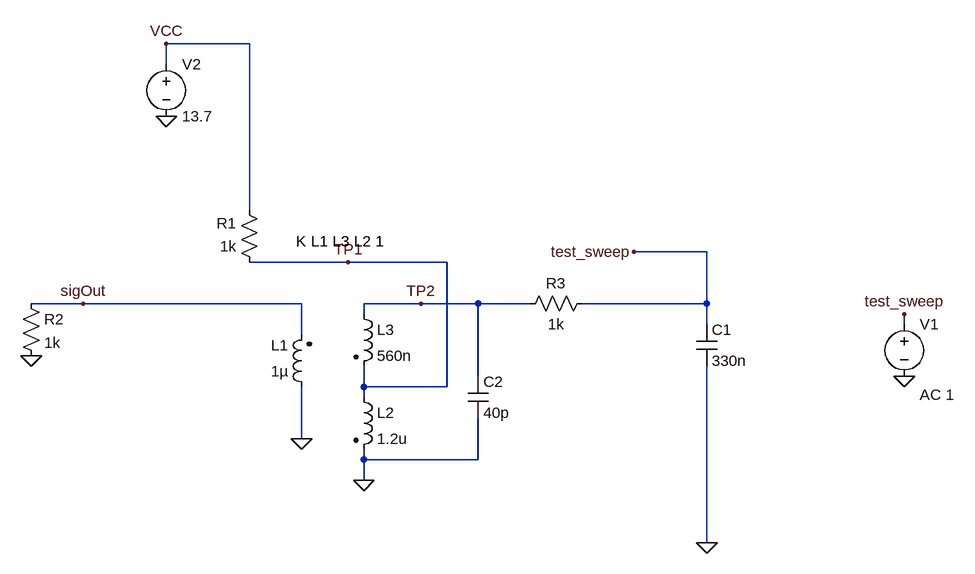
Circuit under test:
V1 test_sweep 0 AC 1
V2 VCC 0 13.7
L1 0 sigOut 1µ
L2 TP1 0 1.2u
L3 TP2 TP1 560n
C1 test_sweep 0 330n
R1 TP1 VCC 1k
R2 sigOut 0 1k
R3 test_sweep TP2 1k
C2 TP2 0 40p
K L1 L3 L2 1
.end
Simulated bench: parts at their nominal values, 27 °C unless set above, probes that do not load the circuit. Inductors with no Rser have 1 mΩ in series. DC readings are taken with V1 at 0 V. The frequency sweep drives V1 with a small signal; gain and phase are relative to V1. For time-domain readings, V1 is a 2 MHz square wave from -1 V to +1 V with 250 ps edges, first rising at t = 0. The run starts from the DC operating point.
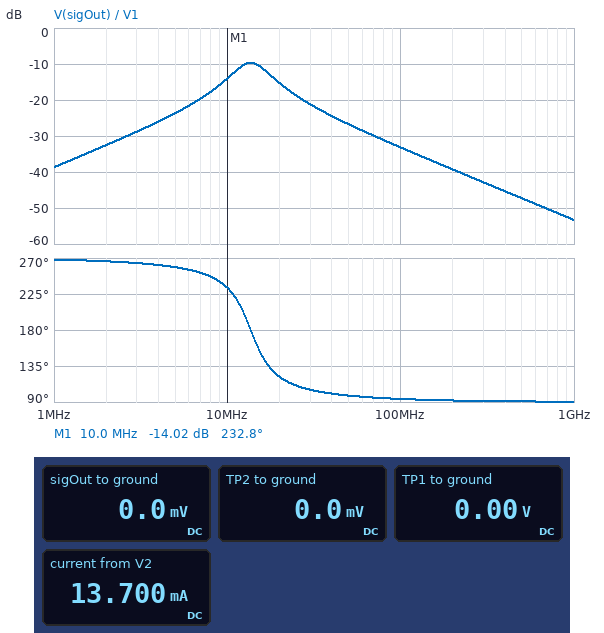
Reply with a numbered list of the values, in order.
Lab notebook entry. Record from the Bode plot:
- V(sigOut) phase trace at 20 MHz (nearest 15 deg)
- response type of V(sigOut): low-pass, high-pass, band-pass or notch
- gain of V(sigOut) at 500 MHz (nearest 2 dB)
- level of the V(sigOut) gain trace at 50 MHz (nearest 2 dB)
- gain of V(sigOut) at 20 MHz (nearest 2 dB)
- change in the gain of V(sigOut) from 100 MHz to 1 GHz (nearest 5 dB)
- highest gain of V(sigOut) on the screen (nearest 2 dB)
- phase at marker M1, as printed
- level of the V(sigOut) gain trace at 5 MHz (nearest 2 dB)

1. 120 deg
2. band-pass
3. -48 dB
4. -26 dB
5. -16 dB
6. -20 dB
7. -10 dB
8. 232.8 deg
9. -24 dB
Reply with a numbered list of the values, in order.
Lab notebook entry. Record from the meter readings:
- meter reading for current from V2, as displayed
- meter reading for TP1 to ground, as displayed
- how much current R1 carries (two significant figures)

1. 13.700 mA
2. 0.00 V
3. 14 mA
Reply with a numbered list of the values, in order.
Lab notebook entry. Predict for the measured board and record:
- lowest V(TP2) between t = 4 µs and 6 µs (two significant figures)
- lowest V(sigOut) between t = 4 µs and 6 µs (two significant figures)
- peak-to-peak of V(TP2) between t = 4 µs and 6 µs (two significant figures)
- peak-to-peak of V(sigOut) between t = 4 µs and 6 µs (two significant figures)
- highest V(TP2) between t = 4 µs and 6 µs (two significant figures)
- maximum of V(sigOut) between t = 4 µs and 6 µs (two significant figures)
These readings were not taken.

1. -420 mV
2. -230 mV
3. 840 mV
4. 460 mV
5. 420 mV
6. 230 mV
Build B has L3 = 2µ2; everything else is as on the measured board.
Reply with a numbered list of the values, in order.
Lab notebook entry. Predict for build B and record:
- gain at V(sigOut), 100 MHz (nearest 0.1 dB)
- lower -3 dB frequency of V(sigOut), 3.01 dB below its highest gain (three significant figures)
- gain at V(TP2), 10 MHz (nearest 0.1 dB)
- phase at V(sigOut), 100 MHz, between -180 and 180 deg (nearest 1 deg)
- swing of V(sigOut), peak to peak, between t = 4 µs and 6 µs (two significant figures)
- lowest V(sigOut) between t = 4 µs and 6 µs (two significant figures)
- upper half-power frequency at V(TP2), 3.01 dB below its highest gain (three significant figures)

1. -36.2 dB
2. 7.46 MHz
3. -2.5 dB
4. 93 deg
5. 440 mV
6. -220 mV
7. 12.8 MHz
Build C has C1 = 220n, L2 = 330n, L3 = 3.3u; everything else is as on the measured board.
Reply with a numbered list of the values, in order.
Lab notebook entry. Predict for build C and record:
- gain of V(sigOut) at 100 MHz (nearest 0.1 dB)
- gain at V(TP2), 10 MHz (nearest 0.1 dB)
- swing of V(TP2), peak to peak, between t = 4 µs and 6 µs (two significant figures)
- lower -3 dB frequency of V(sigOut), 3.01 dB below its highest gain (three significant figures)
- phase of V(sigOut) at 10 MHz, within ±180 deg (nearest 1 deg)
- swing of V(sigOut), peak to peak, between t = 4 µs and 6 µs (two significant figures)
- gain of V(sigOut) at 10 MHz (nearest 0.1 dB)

1. -35.5 dB
2. -2.0 dB
3. 1.1 V
4. 8.35 MHz
5. -168 deg
6. 470 mV
7. -9.6 dB
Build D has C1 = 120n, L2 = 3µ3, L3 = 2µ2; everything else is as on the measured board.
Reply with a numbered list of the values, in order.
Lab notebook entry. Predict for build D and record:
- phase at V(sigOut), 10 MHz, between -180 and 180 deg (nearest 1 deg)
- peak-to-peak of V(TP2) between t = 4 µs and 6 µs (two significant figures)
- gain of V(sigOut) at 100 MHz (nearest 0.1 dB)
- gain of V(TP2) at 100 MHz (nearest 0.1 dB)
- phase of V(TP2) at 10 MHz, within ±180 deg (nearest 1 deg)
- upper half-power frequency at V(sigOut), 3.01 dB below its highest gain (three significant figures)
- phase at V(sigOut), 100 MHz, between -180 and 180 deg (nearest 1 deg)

1. 143 deg
2. 1.3 V
3. -38.3 dB
4. -28.0 dB
5. -37 deg
6. 10.9 MHz
7. 93 deg
